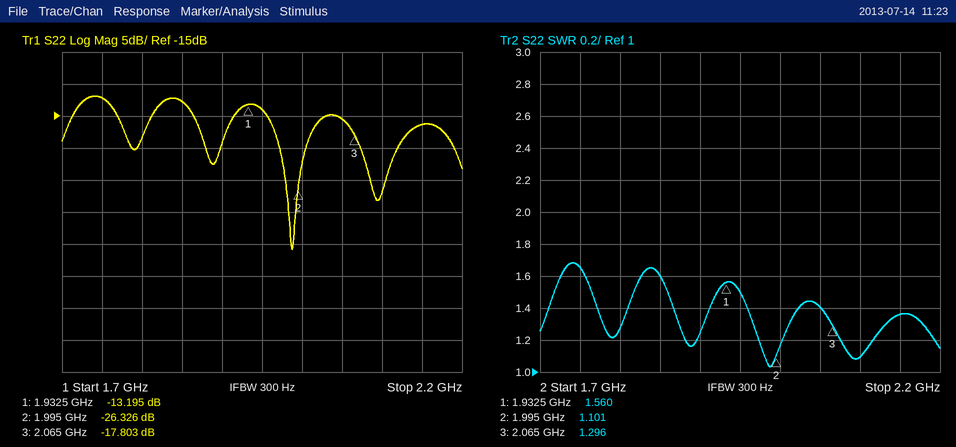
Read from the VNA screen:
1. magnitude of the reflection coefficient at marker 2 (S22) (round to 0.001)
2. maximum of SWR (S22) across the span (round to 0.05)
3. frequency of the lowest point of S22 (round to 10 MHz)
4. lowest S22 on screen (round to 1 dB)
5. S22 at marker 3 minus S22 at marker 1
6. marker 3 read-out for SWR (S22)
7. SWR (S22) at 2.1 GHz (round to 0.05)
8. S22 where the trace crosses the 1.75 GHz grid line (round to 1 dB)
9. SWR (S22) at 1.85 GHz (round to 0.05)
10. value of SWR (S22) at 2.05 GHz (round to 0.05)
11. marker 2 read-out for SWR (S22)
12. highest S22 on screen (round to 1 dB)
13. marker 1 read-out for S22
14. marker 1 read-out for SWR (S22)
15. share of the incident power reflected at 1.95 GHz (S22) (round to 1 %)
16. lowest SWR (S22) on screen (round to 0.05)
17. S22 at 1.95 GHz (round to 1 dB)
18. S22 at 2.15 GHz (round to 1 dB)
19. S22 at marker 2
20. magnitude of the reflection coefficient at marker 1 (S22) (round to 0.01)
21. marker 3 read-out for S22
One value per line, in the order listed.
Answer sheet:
0.048
1.70
1.99 GHz
-36 dB
-4.608 dB
1.296
1.10
-12 dB
1.60
1.40
1.101
-12 dB
-13.195 dB
1.560
4 %
1.05
-14 dB
-16 dB
-26.326 dB
0.22
-17.803 dB
